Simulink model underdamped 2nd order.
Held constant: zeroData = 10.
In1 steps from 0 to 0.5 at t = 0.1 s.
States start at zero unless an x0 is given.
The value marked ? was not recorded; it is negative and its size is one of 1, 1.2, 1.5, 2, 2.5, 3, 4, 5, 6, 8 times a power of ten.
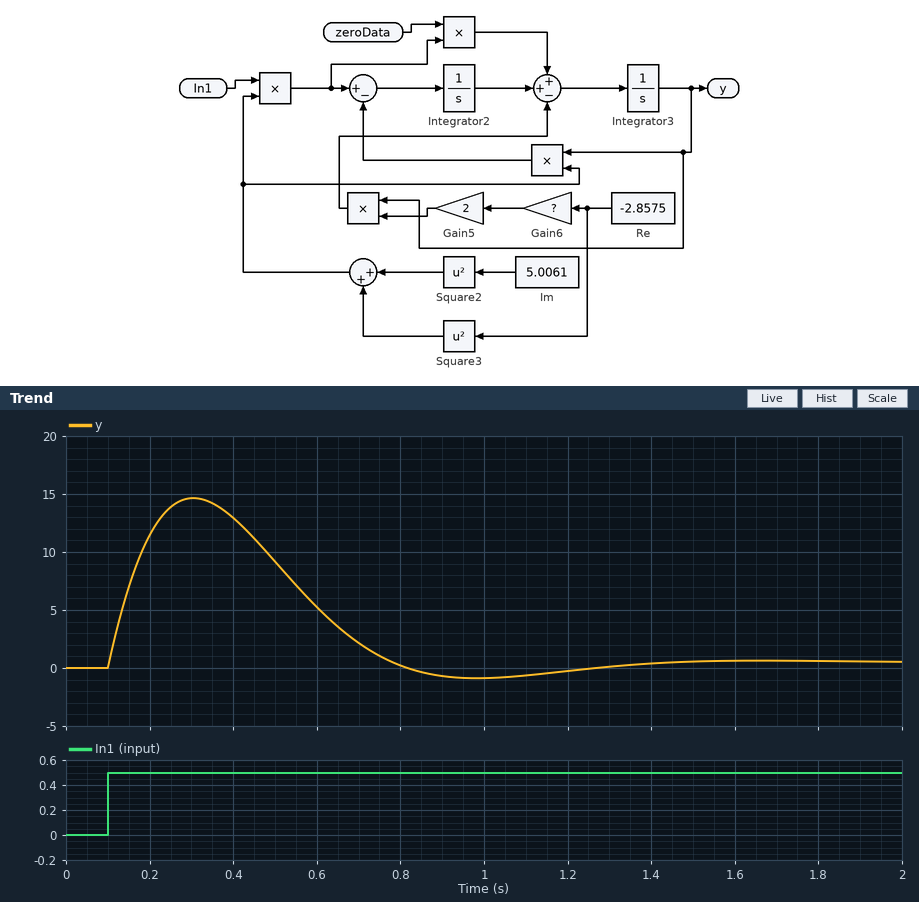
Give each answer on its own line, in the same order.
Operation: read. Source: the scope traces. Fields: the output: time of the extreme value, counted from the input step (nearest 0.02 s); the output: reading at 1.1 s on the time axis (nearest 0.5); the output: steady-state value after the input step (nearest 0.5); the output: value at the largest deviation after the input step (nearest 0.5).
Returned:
0.20 s
-0.5
0.5
14.5
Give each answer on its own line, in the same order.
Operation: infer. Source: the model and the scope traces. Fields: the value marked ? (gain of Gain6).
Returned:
-1.2
